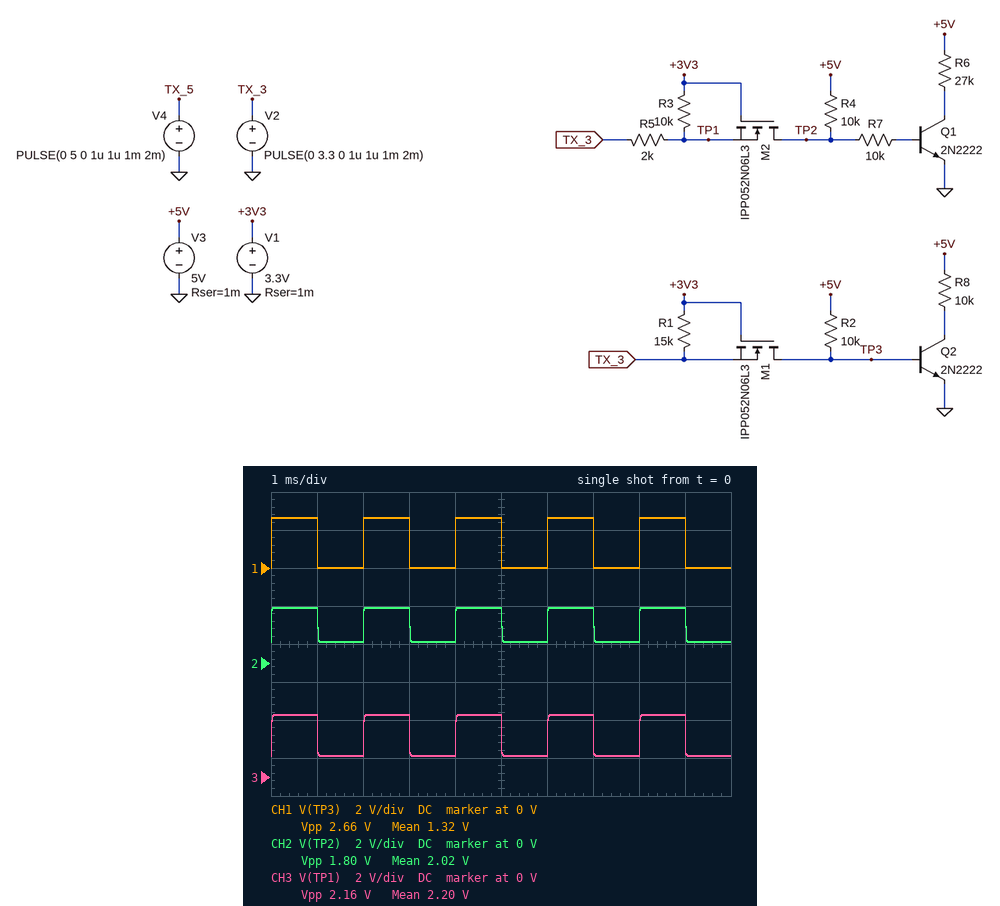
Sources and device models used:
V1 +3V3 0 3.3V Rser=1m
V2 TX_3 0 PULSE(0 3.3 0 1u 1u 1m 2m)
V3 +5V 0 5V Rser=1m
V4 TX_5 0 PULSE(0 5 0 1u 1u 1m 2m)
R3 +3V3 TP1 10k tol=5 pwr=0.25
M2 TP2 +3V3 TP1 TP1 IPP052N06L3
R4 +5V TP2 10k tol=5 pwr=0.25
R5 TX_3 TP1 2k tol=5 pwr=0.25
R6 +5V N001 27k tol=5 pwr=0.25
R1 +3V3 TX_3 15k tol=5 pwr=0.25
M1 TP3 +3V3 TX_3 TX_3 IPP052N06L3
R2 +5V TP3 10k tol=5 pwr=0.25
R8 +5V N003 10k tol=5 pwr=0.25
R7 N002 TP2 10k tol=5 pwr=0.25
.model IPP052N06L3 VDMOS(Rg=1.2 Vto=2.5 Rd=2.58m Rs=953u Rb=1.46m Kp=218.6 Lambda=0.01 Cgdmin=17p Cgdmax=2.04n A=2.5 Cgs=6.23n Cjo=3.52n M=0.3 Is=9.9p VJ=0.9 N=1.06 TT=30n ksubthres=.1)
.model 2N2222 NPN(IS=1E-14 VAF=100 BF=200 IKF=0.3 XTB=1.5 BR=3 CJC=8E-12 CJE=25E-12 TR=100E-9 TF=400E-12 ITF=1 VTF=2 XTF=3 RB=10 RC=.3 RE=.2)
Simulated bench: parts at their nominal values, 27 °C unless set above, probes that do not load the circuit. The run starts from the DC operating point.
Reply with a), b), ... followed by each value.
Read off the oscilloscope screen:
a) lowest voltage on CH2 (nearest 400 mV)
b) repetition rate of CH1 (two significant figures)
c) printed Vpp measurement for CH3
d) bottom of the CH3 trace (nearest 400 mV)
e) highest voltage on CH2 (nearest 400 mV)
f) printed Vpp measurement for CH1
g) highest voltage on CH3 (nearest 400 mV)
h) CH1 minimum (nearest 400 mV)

a) 1.2 V
b) 500 Hz
c) 2.16 V
d) 1.2 V
e) 2.8 V
f) 2.66 V
g) 3.2 V
h) 0 V
